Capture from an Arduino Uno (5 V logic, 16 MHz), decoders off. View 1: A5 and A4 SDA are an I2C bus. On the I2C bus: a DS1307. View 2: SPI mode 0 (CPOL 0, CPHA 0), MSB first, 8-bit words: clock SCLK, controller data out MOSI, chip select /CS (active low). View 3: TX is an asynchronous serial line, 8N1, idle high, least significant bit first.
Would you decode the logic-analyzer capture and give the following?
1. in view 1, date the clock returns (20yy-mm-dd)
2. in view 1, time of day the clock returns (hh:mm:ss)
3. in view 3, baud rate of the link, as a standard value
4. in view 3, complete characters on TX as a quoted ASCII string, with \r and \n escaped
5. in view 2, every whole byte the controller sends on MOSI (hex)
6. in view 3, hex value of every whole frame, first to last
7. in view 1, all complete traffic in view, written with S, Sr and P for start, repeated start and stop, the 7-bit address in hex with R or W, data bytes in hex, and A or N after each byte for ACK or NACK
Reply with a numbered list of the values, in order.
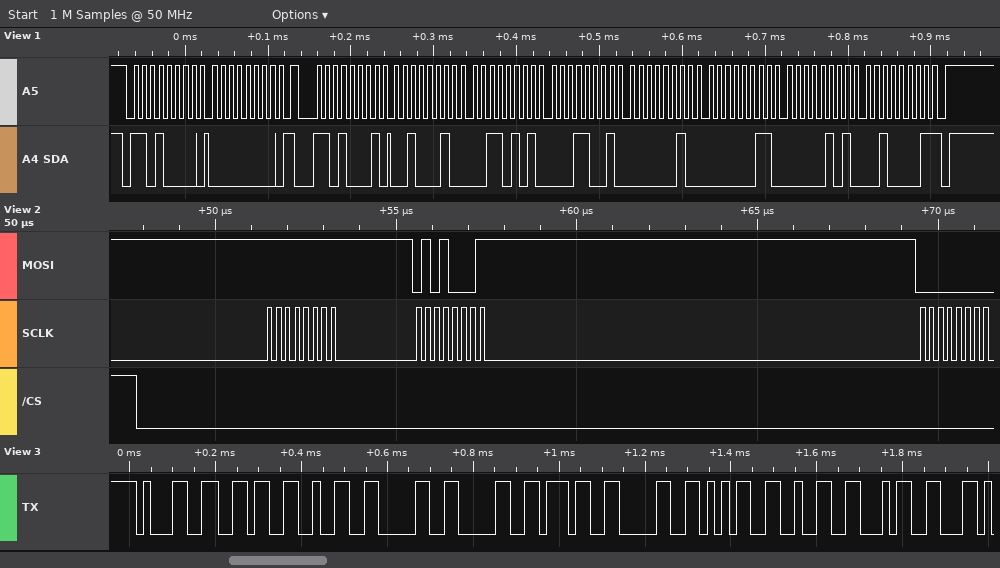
1. 2021-05-03
2. 19:35:22
3. 57600 baud
4. "1620070524"
5. 0xFF 0x51 0x00
6. 0x31 0x36 0x32 0x30 0x30 0x37 0x30 0x35 0x32 0x34
7. S 68W A 00 A Sr 68R A 22 A 35 A 19 A 02 A 03 A 05 A 21 N P
